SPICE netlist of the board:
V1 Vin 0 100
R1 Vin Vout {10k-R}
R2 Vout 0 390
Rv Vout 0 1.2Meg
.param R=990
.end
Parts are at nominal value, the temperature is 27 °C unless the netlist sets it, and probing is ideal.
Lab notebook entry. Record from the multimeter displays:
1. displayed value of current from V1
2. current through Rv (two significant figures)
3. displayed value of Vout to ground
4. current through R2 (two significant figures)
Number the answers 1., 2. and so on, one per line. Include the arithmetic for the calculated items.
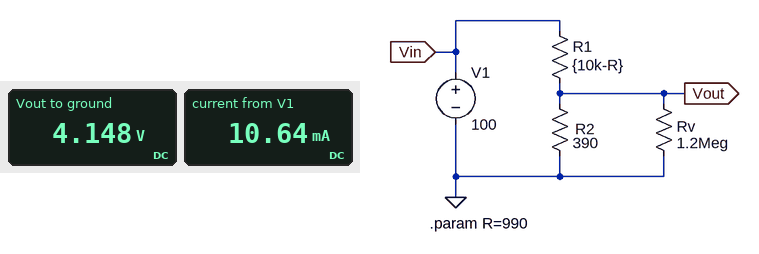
1. 10.64 mA
2. (4.148 V) / 1.2 MΩ = 3.5 µA
3. 4.148 V
4. (4.148 V) / 390 Ω = 11 mA
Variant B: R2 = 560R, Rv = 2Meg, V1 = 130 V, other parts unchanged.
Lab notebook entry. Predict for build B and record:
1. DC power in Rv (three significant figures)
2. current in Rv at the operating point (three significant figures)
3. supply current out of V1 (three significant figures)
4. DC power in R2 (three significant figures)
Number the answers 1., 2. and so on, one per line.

1. 28.9 µW
2. 3.80 µA
3. 13.6 mA
4. 103 mW
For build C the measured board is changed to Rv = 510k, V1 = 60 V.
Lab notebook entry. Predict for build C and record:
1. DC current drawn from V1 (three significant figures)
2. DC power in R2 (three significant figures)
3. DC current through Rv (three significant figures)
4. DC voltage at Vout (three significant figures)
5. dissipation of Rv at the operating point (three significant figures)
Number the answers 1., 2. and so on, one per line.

1. 6.38 mA
2. 15.9 mW
3. 4.88 µA
4. 2.49 V
5. 12.1 µW
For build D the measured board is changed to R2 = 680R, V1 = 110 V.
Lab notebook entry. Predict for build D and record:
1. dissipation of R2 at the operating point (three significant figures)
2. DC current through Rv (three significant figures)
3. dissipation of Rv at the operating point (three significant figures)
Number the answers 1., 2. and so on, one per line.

1. 87.5 mW
2. 6.43 µA
3. 49.6 µW
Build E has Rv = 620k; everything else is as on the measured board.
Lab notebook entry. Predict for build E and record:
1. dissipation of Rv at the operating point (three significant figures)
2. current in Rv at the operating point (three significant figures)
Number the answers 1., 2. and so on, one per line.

1. 27.7 µW
2. 6.69 µA
